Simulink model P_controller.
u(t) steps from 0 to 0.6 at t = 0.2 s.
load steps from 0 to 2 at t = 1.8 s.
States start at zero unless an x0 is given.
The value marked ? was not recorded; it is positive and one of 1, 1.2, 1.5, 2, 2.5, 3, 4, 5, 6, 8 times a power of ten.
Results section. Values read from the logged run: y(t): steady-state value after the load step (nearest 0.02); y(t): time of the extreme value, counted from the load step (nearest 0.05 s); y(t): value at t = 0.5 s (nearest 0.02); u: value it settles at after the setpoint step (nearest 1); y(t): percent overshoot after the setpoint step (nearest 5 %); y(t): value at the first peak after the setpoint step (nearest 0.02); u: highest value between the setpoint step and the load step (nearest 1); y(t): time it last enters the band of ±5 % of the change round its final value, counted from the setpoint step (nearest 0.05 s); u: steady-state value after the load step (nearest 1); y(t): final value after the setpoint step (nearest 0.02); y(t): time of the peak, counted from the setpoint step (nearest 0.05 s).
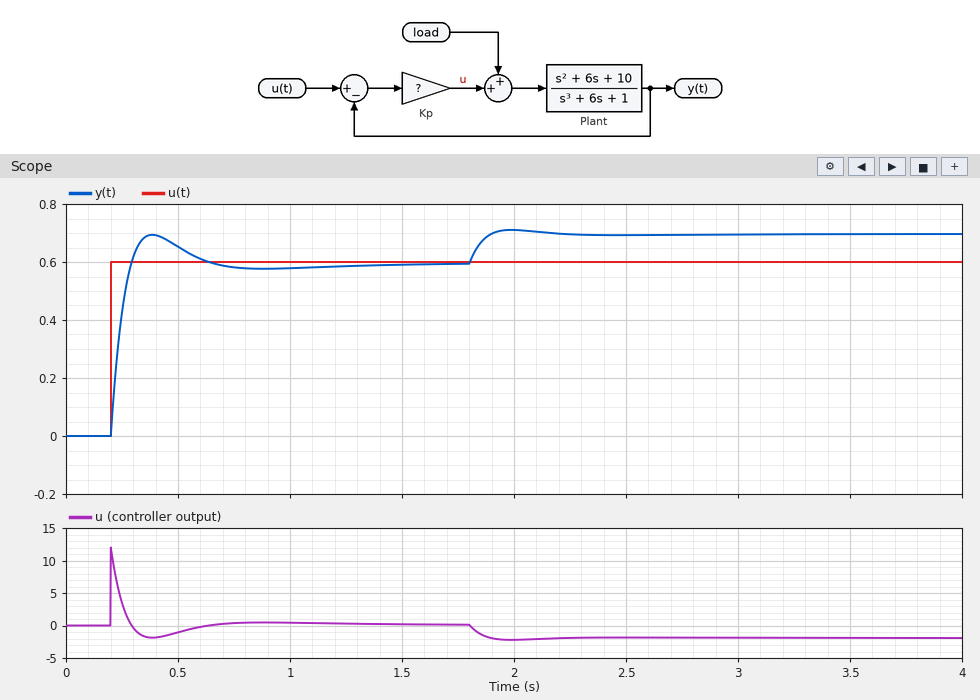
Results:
0.70
0.20 s
0.66
0
15 %
0.70
12
0.35 s
-2
0.60
0.20 s
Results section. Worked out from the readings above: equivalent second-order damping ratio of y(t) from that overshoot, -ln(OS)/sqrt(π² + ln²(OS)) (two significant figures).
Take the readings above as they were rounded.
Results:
0.52
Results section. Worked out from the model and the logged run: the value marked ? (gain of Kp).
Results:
20
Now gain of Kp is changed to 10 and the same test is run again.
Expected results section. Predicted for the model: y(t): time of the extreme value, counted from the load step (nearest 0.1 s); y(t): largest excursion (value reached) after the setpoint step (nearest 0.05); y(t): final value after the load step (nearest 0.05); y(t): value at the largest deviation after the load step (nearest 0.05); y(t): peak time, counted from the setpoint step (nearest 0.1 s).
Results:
0.3 s
0.75
0.80
0.85
0.3 s
